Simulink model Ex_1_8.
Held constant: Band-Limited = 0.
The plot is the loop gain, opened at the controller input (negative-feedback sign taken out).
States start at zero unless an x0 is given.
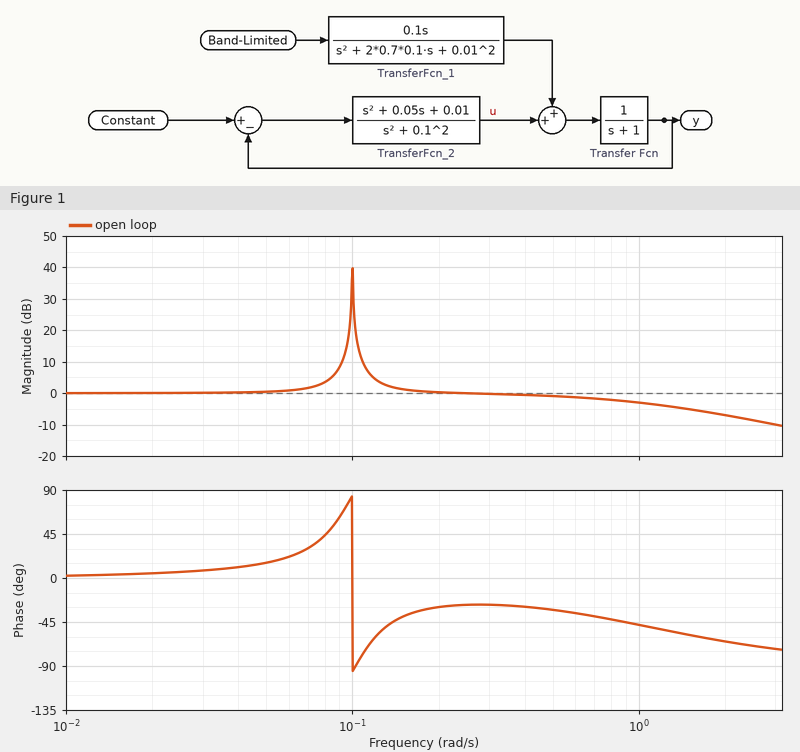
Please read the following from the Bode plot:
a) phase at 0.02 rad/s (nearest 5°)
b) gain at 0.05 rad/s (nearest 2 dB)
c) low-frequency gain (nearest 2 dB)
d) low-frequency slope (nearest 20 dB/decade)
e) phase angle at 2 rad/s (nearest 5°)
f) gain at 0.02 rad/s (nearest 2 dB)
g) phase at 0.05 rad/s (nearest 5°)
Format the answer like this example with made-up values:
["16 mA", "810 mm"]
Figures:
["5°", "0 dB", "0 dB", "0 dB/decade", "-65°", "0 dB", "15°"]
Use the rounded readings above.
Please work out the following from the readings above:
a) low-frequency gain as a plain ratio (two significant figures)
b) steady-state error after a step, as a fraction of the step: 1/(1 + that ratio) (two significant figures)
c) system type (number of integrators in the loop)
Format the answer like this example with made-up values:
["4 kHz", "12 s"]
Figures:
["1.0", "0.50", "0"]
